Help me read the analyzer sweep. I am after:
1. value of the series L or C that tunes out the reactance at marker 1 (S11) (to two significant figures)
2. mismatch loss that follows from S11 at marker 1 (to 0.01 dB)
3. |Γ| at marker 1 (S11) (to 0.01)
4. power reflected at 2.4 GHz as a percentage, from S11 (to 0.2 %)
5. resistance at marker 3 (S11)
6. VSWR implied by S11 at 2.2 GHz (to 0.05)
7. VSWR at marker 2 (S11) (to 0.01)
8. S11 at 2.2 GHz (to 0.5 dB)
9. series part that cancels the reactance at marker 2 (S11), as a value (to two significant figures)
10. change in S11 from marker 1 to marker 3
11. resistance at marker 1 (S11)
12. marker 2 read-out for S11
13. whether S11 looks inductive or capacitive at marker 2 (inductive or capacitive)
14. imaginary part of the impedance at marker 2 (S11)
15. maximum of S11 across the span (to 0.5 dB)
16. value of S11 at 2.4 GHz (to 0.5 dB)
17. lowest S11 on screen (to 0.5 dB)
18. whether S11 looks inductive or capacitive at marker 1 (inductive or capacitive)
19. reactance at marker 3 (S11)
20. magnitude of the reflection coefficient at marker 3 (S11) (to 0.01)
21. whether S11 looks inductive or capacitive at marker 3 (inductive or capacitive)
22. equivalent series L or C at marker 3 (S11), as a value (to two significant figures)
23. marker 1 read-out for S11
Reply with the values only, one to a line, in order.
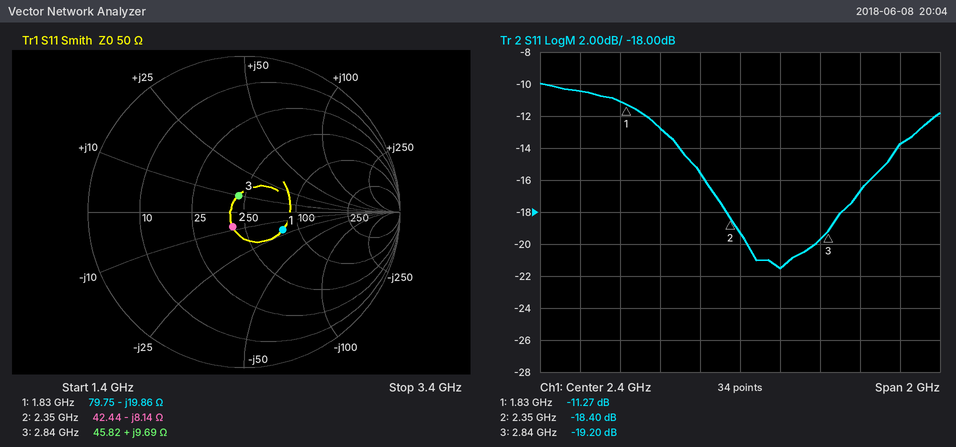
1.7 nH
0.34 dB
0.27
1.2 %
45.82 Ω
1.40
1.27
-15.5 dB
550 pH
-7.93 dB
79.75 Ω
-18.40 dB
capacitive
-8.14 Ω
-10.0 dB
-19.5 dB
-21.5 dB
capacitive
+9.69 Ω
0.11
inductive
540 pH
-11.27 dB
